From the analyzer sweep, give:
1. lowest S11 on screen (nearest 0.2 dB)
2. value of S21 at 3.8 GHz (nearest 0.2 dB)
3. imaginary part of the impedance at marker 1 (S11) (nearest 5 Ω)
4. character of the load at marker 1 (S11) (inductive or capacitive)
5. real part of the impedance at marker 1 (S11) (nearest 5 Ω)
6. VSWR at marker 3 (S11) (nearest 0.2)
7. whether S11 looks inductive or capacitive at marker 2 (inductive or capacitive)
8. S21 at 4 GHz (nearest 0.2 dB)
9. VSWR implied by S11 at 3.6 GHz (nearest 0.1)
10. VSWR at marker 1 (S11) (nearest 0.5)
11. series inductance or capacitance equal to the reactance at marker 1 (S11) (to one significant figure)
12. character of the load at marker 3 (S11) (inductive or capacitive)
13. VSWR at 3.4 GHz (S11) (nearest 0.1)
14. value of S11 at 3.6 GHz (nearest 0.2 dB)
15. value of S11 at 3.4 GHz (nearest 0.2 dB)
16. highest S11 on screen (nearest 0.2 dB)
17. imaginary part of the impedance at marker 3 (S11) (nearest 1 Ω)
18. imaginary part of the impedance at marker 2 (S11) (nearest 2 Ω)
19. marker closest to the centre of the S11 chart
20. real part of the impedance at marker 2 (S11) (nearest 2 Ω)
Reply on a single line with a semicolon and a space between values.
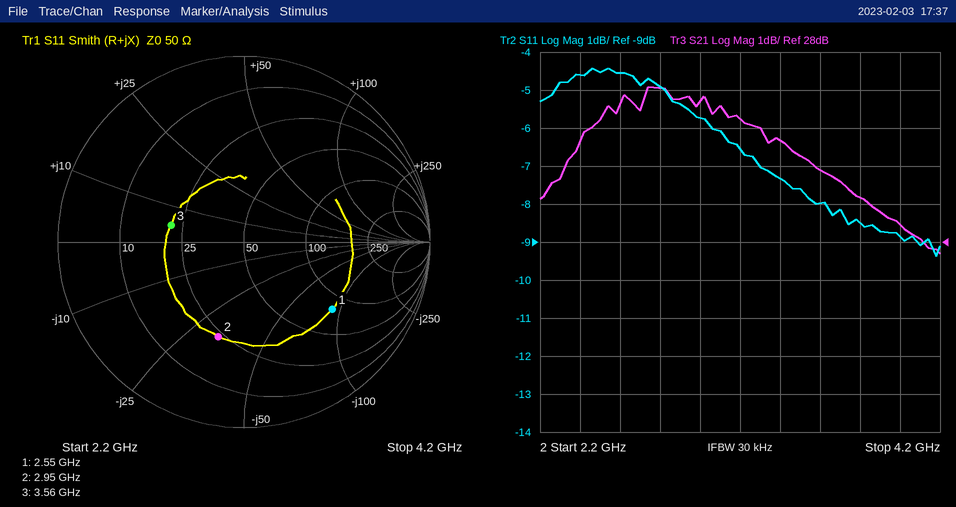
-9.4 dB; 29.2 dB; -90 Ω; capacitive; 80 Ω; 2.4; capacitive; 28.4 dB; 2.3; 4.0; 700 fF; inductive; 2.5; -8.0 dB; -7.4 dB; -4.4 dB; +5 Ω; -32 Ω; marker 3; 24 Ω
